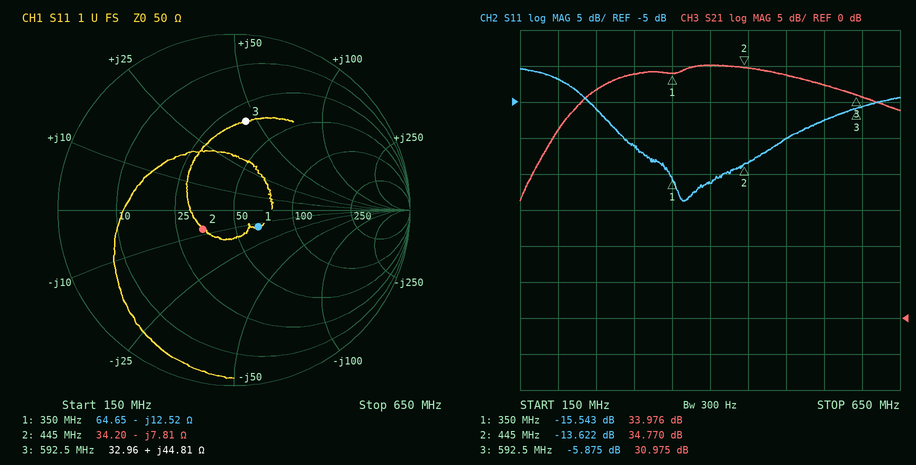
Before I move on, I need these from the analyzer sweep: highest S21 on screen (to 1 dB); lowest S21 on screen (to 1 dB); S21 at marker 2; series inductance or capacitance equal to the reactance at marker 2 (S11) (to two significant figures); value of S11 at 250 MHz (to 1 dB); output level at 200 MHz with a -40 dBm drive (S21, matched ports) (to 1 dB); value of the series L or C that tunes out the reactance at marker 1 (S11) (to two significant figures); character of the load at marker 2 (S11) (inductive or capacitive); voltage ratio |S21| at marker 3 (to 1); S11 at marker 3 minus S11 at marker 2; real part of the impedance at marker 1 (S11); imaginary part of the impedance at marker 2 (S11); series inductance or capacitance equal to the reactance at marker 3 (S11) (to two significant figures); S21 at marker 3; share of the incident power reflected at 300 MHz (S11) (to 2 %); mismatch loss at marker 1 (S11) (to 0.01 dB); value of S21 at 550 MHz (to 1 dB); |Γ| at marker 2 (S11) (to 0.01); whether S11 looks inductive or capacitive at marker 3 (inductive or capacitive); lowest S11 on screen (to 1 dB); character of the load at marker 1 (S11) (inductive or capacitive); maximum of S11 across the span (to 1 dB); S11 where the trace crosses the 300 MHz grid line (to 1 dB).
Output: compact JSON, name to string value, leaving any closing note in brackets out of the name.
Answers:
{"highest S21 on screen": "35 dB", "lowest S21 on screen": "16 dB", "S21 at marker 2": "34.770 dB", "series inductance or capacitance equal to the reactance at marker 2 (S11)": "46 pF", "value of S11 at 250 MHz": "-6 dB", "output level at 200 MHz with a -40 dBm drive (S21, matched ports)": "-14 dBm", "value of the series L or C that tunes out the reactance at marker 1 (S11)": "5.7 nH", "character of the load at marker 2 (S11)": "capacitive", "voltage ratio |S21| at marker 3": "35", "S11 at marker 3 minus S11 at marker 2": "7.747 dB", "real part of the impedance at marker 1": "64.65 Ω", "imaginary part of the impedance at marker 2": "-7.81 Ω", "series inductance or capacitance equal to the reactance at marker 3 (S11)": "12 nH", "S21 at marker 3": "30.975 dB", "share of the incident power reflected at 300 MHz (S11)": "8 %", "mismatch loss at marker 1 (S11)": "0.12 dB", "value of S21 at 550 MHz": "32 dB", "|Γ| at marker 2 (S11)": "0.21", "whether S11 looks inductive or capacitive at marker 3": "inductive", "lowest S11 on screen": "-19 dB", "character of the load at marker 1 (S11)": "capacitive", "maximum of S11 across the span": "0 dB", "S11 where the trace crosses the 300 MHz grid line": "-11 dB"}
